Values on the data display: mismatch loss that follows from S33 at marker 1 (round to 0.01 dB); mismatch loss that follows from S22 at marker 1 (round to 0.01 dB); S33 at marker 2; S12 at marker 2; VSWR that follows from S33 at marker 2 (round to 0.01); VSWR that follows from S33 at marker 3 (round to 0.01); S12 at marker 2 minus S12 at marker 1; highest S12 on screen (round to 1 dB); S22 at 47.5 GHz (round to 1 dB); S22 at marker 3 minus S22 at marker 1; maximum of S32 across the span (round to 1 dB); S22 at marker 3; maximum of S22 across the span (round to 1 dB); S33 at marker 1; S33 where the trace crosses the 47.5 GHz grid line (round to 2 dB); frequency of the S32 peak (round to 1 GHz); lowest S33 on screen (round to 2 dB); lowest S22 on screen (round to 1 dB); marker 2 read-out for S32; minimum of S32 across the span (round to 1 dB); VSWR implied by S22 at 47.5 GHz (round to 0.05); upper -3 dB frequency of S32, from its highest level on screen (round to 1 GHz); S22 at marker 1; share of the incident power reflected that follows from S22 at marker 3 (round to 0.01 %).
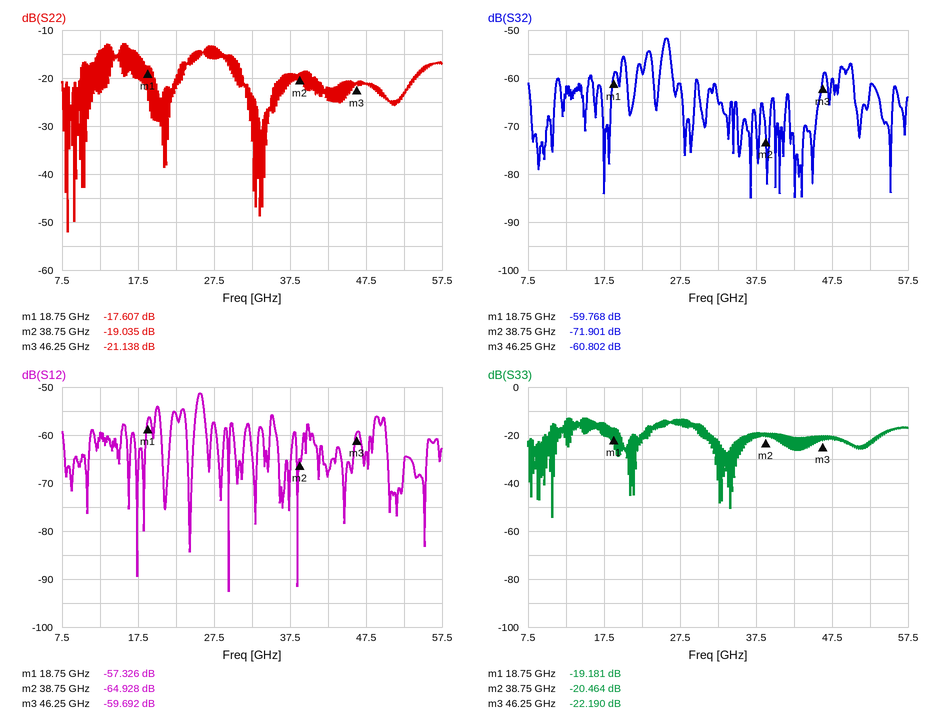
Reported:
0.05 dB
0.08 dB
-20.464 dB
-64.928 dB
1.21
1.17
-7.602 dB
-51 dB
-21 dB
-3.531 dB
-52 dB
-21.138 dB
-13 dB
-19.181 dB
-22 dB
26 GHz
-54 dB
-52 dB
-71.901 dB
-85 dB
1.20
26 GHz
-17.607 dB
0.77 %
